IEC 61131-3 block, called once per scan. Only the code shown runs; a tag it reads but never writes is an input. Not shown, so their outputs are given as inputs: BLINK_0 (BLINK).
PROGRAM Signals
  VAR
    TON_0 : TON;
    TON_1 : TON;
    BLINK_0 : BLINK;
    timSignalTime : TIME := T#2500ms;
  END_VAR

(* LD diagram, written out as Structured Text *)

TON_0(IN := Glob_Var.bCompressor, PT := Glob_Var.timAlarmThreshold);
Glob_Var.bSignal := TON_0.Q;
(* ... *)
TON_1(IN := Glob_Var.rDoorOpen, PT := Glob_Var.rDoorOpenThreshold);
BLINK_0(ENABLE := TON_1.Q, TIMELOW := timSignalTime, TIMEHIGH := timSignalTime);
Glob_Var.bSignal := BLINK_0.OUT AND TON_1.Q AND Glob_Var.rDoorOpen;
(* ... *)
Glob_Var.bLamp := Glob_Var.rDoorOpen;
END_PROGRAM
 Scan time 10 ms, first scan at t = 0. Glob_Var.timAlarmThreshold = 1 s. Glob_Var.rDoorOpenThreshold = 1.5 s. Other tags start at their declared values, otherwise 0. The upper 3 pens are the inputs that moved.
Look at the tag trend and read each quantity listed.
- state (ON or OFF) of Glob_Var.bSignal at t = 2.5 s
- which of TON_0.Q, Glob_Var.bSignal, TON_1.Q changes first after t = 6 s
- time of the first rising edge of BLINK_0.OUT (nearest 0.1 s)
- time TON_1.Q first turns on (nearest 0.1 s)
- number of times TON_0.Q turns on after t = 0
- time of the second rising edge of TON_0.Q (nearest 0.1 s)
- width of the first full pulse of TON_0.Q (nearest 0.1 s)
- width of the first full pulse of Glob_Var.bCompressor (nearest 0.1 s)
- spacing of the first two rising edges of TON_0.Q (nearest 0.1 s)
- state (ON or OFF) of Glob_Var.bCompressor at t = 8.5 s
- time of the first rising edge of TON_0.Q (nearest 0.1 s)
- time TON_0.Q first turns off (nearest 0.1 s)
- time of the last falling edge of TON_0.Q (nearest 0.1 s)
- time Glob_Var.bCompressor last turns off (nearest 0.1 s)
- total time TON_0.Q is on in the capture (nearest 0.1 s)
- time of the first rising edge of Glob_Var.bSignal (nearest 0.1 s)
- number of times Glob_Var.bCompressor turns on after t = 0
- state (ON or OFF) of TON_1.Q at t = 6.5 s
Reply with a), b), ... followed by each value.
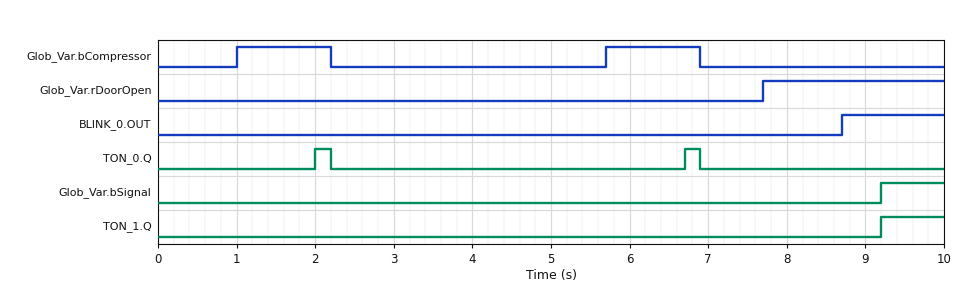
a) OFF
b) TON_0.Q
c) 8.7 s
d) 9.2 s
e) 2
f) 6.7 s
g) 0.2 s
h) 1.2 s
i) 4.7 s
j) OFF
k) 2.0 s
l) 2.2 s
m) 6.9 s
n) 6.9 s
o) 0.4 s
p) 9.2 s
q) 2
r) OFF
